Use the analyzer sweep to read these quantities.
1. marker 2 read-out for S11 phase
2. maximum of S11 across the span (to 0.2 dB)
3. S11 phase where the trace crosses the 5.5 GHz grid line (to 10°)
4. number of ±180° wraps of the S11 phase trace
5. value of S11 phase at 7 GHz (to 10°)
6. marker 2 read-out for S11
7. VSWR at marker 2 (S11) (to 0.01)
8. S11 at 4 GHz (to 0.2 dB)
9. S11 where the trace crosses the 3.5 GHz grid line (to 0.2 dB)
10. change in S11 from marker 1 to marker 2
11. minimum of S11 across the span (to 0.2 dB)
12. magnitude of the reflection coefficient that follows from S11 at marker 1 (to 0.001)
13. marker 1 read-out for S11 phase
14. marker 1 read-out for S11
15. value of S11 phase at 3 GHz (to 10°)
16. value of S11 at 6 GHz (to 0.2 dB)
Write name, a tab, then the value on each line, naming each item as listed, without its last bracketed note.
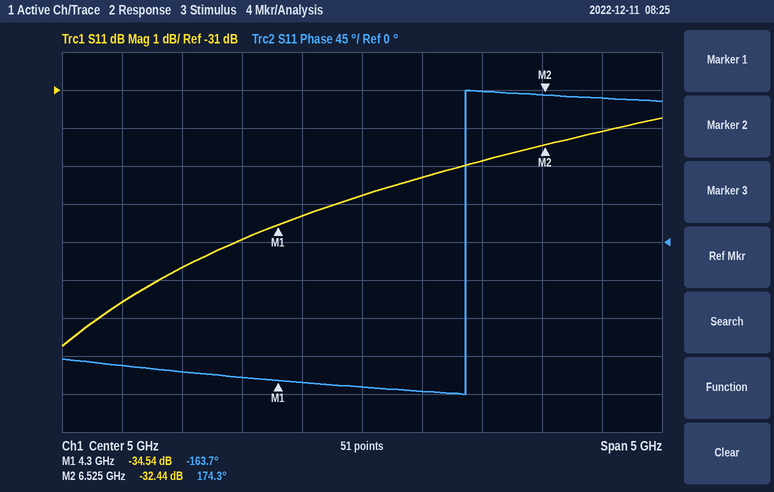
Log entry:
marker 2 read-out for S11 phase	174.3°
maximum of S11 across the span	-31.8 dB
S11 phase where the trace crosses the 5.5 GHz grid line	-180°
number of ±180° wraps of the S11 phase trace	1
value of S11 phase at 7 GHz	170°
marker 2 read-out for S11	-32.44 dB
VSWR at marker 2 (S11)	1.05
S11 at 4 GHz	-35.0 dB
S11 where the trace crosses the 3.5 GHz grid line	-35.6 dB
change in S11 from marker 1 to marker 2	2.10 dB
minimum of S11 across the span	-37.8 dB
magnitude of the reflection coefficient that follows from S11 at marker 1	0.019
marker 1 read-out for S11 phase	-163.7°
marker 1 read-out for S11	-34.54 dB
value of S11 phase at 3 GHz	-150°
value of S11 at 6 GHz	-32.8 dB
